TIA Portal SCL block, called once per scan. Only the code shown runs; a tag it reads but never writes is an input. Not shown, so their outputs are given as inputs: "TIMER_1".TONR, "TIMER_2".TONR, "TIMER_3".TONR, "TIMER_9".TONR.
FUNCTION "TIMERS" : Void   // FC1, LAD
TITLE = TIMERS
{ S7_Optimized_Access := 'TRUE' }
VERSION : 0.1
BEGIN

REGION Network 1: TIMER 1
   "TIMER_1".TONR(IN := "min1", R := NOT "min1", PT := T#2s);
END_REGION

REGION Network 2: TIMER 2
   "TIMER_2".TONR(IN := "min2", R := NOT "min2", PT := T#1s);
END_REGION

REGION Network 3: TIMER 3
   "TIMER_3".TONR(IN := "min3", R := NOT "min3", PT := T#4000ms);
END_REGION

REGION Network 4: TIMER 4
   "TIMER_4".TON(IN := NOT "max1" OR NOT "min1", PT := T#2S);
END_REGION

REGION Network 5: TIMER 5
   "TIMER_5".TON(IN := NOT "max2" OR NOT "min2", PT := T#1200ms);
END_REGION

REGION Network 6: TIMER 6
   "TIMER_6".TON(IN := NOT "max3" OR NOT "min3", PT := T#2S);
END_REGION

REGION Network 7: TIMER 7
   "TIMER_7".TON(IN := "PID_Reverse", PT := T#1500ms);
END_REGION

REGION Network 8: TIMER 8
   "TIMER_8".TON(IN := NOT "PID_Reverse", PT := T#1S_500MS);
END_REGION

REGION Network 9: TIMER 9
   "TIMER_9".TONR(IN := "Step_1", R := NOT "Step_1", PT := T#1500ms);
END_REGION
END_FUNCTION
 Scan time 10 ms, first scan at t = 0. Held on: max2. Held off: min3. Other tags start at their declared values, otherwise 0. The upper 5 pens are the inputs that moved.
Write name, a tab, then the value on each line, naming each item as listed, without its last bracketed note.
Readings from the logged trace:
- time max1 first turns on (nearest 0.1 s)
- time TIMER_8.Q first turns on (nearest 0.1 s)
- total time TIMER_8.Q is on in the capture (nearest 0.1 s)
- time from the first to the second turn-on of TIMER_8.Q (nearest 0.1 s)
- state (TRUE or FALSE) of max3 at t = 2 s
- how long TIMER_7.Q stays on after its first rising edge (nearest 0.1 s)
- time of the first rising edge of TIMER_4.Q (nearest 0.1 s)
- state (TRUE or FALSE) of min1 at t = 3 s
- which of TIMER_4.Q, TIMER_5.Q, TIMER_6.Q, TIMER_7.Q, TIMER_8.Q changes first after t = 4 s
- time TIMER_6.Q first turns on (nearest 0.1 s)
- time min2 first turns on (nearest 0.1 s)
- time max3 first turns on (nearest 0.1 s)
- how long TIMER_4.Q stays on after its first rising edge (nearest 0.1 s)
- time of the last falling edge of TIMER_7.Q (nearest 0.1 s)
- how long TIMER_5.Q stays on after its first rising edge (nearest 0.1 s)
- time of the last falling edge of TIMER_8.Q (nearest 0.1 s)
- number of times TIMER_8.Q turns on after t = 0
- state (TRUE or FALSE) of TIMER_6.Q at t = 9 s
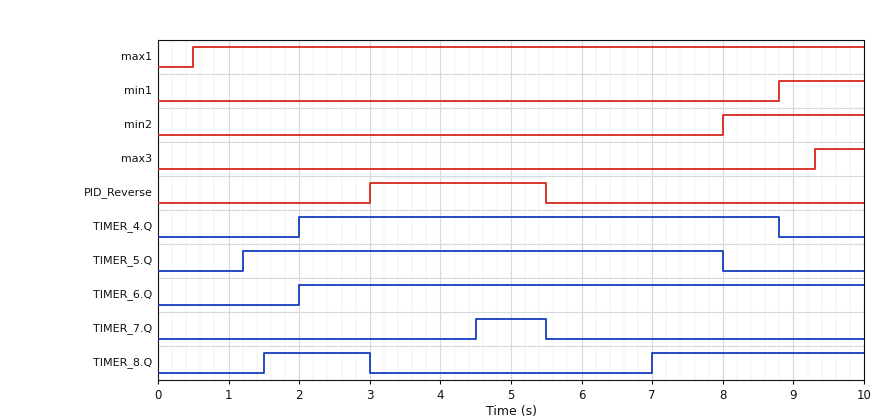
time max1 first turns on	0.5 s
time TIMER_8.Q first turns on	1.5 s
total time TIMER_8.Q is on in the capture	4.5 s
time from the first to the second turn-on of TIMER_8.Q	5.5 s
state (TRUE or FALSE) of max3 at t = 2 s	FALSE
how long TIMER_7.Q stays on after its first rising edge	1.0 s
time of the first rising edge of TIMER_4.Q	2.0 s
state (TRUE or FALSE) of min1 at t = 3 s	FALSE
which of TIMER_4.Q, TIMER_5.Q, TIMER_6.Q, TIMER_7.Q, TIMER_8.Q changes first after t = 4 s	TIMER_7.Q
time TIMER_6.Q first turns on	2.0 s
time min2 first turns on	8.0 s
time max3 first turns on	9.3 s
how long TIMER_4.Q stays on after its first rising edge	6.8 s
time of the last falling edge of TIMER_7.Q	5.5 s
how long TIMER_5.Q stays on after its first rising edge	6.8 s
time of the last falling edge of TIMER_8.Q	3.0 s
number of times TIMER_8.Q turns on after t = 0	2
state (TRUE or FALSE) of TIMER_6.Q at t = 9 s	TRUE
